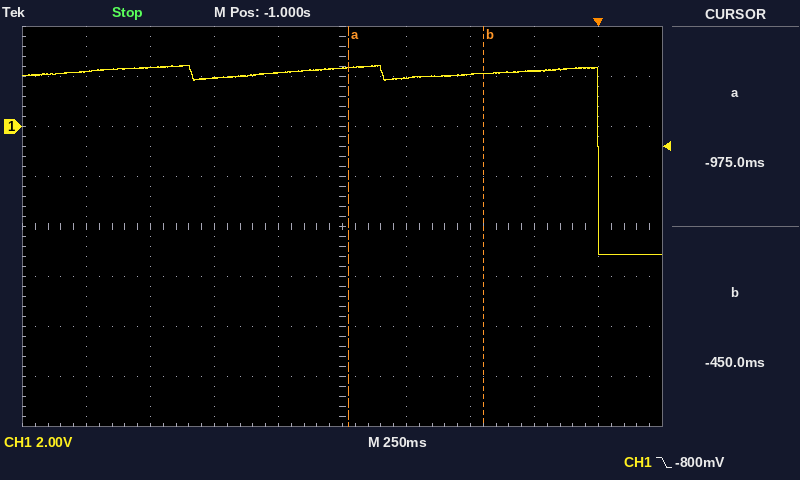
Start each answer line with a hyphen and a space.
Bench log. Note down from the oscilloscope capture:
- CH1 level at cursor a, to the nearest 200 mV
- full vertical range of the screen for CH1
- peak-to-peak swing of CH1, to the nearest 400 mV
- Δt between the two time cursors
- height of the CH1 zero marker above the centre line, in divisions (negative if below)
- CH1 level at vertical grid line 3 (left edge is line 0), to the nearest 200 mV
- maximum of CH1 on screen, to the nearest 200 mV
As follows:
- 2.4 V
- 16 V
- 7.6 V
- 525 ms
- +2.0 div
- 2.0 V
- 2.4 V
